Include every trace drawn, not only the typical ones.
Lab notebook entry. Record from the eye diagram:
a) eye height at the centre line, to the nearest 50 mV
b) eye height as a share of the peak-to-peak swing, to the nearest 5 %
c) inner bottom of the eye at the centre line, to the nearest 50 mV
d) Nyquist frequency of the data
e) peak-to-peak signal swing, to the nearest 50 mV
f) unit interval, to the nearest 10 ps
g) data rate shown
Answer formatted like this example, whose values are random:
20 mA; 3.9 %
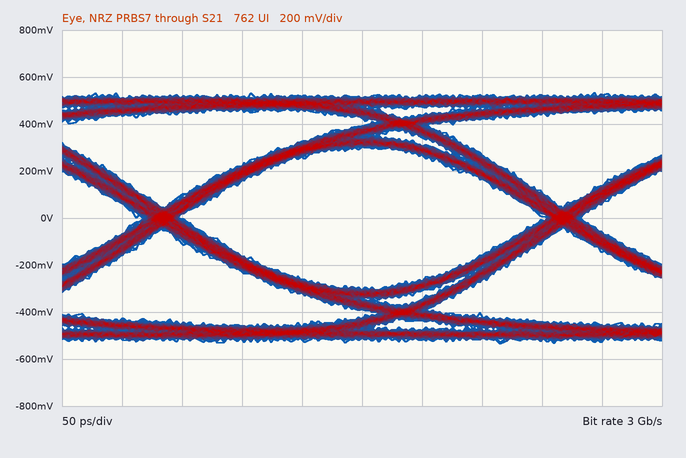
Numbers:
600 mV; 55 %; -300 mV; 1.5 GHz; 1.05 V; 330 ps; 3 Gb/s
